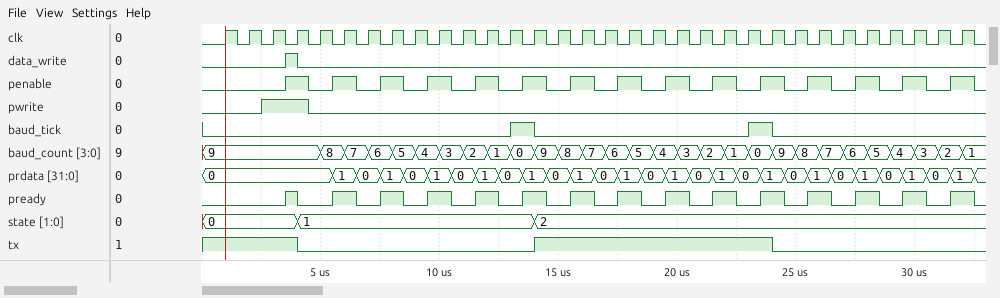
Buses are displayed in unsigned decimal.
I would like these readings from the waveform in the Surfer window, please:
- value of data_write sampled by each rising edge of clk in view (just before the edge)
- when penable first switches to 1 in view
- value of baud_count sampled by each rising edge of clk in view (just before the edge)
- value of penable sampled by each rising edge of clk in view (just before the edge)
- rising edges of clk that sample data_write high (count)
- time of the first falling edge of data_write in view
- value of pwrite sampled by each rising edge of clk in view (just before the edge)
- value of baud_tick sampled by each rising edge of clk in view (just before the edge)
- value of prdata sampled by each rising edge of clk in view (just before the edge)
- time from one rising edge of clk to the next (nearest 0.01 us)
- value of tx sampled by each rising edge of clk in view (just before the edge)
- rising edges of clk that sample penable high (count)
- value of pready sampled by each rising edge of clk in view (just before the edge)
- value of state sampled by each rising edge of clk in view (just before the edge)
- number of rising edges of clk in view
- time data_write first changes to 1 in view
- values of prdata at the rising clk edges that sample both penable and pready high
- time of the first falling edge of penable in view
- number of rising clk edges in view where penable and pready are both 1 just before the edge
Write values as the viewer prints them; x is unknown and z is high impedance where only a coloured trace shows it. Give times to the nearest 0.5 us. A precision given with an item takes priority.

0 0 0 1 0 0 0 0 0 0 0 0 0 0 0 0 0 0 0 0 0 0 0 0 0 0 0 0 0 0 0 0
3.5 us
9, 9, 9, 9, 9, 8, 7, 6, 5, 4, 3, 2, 1, 0, 9, 8, 7, 6, 5, 4, 3, 2, 1, 0, 9, 8, 7, 6, 5, 4, 3, 2
0 0 0 1 0 1 0 1 0 1 0 1 0 1 0 1 0 1 0 1 0 1 0 1 0 1 0 1 0 1 0 1
1
4 us
0 0 1 1 0 0 0 0 0 0 0 0 0 0 0 0 0 0 0 0 0 0 0 0 0 0 0 0 0 0 0 0
0 0 0 0 0 0 0 0 0 0 0 0 0 1 0 0 0 0 0 0 0 0 0 1 0 0 0 0 0 0 0 0
0, 0, 0, 0, 0, 1, 0, 1, 0, 1, 0, 1, 0, 1, 0, 1, 0, 1, 0, 1, 0, 1, 0, 1, 0, 1, 0, 1, 0, 1, 0, 1
1 us
1 1 1 1 0 0 0 0 0 0 0 0 0 0 1 1 1 1 1 1 1 1 1 1 0 0 0 0 0 0 0 0
15
0 0 0 1 0 1 0 1 0 1 0 1 0 1 0 1 0 1 0 1 0 1 0 1 0 1 0 1 0 1 0 1
0, 0, 0, 0, 1, 1, 1, 1, 1, 1, 1, 1, 1, 1, 2, 2, 2, 2, 2, 2, 2, 2, 2, 2, 2, 2, 2, 2, 2, 2, 2, 2
32
3.5 us
0, 1, 1, 1, 1, 1, 1, 1, 1, 1, 1, 1, 1, 1, 1
4.5 us
15
